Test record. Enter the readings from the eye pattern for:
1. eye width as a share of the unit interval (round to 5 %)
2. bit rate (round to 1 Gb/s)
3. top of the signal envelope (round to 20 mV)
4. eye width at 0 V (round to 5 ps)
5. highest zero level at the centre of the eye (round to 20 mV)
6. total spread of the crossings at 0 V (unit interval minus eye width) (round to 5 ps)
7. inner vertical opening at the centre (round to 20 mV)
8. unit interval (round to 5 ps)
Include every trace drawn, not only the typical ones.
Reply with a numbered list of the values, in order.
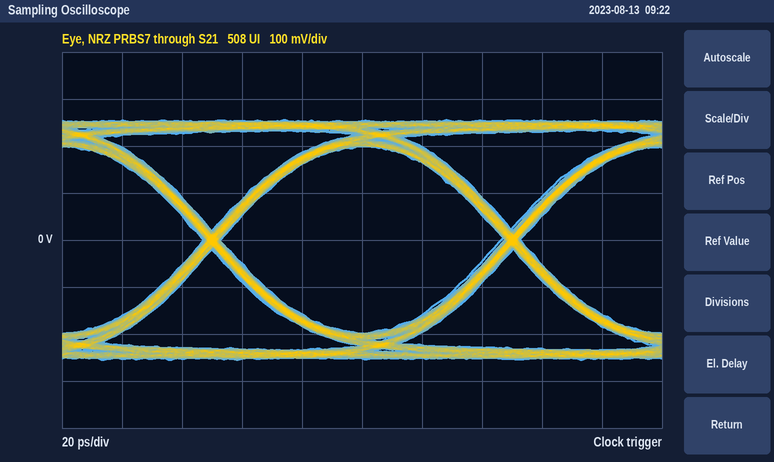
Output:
1. 95 %
2. 10 Gb/s
3. 260 mV
4. 95 ps
5. -200 mV
6. 5 ps
7. 400 mV
8. 100 ps
